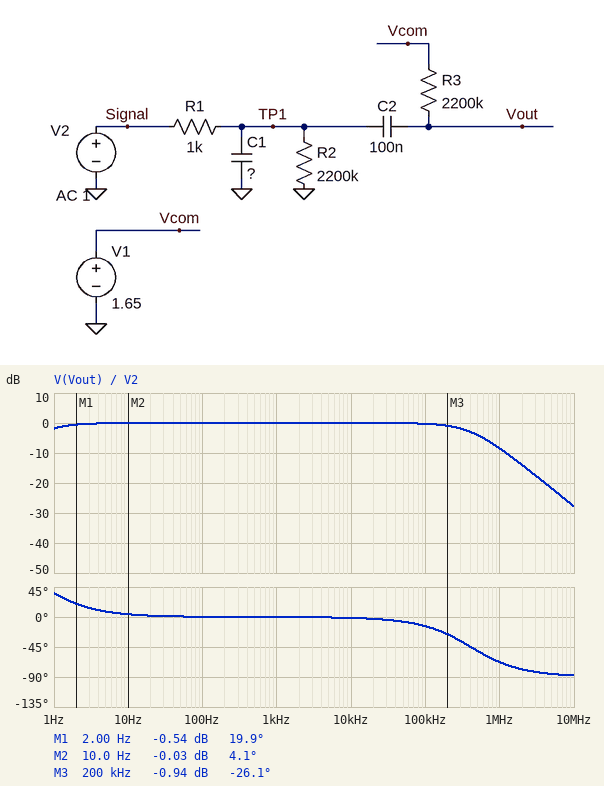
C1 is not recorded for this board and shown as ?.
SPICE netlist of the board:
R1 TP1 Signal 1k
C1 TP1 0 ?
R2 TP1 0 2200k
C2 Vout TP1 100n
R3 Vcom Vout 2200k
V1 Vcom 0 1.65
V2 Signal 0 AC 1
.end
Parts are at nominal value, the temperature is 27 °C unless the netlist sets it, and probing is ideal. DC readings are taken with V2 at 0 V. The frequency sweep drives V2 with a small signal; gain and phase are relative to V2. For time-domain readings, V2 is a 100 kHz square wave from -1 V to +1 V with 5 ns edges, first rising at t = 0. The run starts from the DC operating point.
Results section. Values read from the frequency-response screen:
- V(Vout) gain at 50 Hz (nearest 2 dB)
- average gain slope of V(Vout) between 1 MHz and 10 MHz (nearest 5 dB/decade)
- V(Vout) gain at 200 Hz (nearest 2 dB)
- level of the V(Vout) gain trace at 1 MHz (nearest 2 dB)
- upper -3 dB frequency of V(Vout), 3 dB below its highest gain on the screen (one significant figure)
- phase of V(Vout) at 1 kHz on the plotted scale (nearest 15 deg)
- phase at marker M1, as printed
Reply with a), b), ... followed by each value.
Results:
a) 0 dB
b) -20 dB/decade
c) 0 dB
d) -8 dB
e) 400 kHz
f) 0 deg
g) 19.9 deg
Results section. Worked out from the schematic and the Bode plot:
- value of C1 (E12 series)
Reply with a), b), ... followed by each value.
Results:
a) 390 pF
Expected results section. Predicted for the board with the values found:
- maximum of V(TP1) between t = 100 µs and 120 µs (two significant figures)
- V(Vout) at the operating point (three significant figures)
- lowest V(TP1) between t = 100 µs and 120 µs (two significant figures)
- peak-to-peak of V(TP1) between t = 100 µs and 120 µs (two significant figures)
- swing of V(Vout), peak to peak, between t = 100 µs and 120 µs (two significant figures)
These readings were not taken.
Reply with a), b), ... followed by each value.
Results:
a) 1.0 V
b) 1.65 V
c) -1.0 V
d) 2.0 V
e) 2.0 V
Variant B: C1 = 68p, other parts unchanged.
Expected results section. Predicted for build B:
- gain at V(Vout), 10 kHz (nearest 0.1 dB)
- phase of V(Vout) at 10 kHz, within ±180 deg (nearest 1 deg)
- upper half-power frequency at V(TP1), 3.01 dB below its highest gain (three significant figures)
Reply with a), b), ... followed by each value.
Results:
a) 0 dB
b) 0 deg
c) 2.34 MHz
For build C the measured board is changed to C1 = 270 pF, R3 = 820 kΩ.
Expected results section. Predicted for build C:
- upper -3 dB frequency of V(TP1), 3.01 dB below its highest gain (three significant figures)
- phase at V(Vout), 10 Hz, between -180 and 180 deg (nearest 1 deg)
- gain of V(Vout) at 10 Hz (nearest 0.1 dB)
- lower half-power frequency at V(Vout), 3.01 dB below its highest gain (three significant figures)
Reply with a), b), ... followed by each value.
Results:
a) 589 kHz
b) 11 deg
c) -0.2 dB
d) 1.94 Hz
